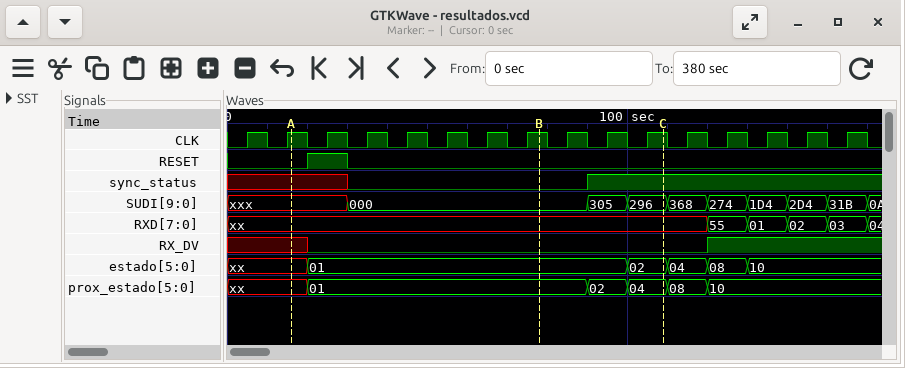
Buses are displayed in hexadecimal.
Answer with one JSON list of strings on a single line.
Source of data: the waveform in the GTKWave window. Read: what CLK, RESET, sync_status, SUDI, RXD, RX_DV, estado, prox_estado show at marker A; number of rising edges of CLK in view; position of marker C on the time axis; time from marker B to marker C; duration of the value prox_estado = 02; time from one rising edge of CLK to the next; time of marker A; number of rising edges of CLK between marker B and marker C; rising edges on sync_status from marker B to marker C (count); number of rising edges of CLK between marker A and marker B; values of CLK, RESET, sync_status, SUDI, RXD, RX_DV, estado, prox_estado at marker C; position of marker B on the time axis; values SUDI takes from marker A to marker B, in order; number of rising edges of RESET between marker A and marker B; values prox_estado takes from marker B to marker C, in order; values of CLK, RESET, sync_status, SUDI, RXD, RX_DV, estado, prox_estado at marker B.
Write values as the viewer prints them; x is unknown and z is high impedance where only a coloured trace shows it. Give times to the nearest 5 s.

["CLK=1, RESET=0, sync_status=x, SUDI=xxx, RXD=xx, RX_DV=x, estado=xx, prox_estado=xx", "16", "110 s", "30 s", "10 s", "10 s", "15 s", "3", "1", "6", "CLK=1, RESET=0, sync_status=1, SUDI=296, RXD=xx, RX_DV=0, estado=02, prox_estado=04", "80 s", "xxx, 000", "1", "01, 02, 04", "CLK=1, RESET=0, sync_status=0, SUDI=000, RXD=xx, RX_DV=0, estado=01, prox_estado=01"]
